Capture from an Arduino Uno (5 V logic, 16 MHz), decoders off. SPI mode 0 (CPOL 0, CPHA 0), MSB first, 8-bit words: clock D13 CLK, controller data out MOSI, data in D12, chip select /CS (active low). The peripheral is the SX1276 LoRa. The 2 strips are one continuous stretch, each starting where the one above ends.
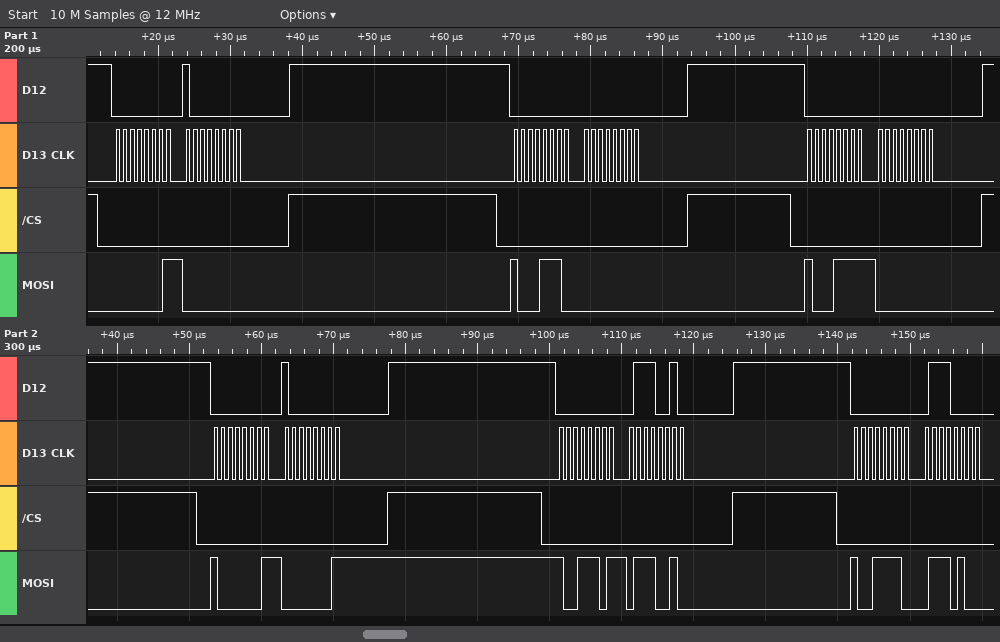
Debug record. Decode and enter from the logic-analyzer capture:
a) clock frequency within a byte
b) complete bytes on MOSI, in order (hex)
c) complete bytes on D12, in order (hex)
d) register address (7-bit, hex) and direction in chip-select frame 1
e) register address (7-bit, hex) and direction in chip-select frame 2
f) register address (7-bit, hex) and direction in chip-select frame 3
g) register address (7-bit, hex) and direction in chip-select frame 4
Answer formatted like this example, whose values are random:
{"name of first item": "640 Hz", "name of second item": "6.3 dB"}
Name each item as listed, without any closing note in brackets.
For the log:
{"clock frequency within a byte": "1 MHz", "complete bytes on MOSI, in order": "01 00 8E 00 8F 00 81 01 9D 72 9E 74", "complete bytes on D12, in order": "00 80 00 00 00 00 00 80 00 72 00 70", "register address (7-bit, hex) and direction in chip-select frame 1": "0x01 read", "register address (7-bit, hex) and direction in chip-select frame 2": "0x0E write", "register address (7-bit, hex) and direction in chip-select frame 3": "0x0F write", "register address (7-bit, hex) and direction in chip-select frame 4": "0x01 write"}
